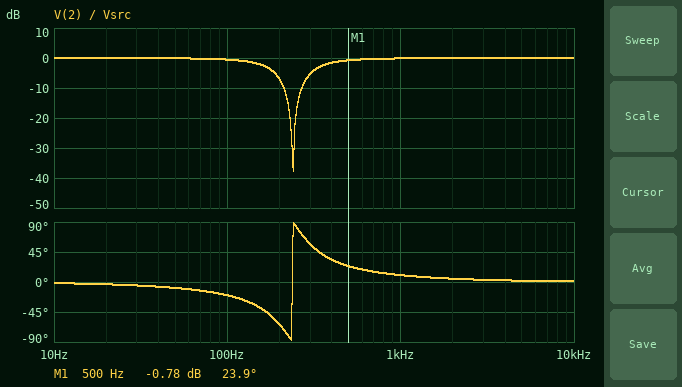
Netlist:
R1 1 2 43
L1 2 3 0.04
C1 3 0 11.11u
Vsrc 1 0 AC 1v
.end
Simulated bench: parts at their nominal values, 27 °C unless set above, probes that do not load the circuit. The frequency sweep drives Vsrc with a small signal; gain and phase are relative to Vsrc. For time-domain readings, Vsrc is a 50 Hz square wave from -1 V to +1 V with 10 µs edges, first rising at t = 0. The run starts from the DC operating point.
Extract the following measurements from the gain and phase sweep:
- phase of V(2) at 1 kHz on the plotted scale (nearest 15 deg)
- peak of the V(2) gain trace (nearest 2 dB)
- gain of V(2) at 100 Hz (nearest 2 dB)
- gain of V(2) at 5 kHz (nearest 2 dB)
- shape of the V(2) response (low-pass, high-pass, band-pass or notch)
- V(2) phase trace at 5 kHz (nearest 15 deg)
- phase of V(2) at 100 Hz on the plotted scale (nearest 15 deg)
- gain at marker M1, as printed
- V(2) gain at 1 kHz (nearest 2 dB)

15 deg
0 dB
0 dB
0 dB
notch
0 deg
-15 deg
-0.78 dB
0 dB
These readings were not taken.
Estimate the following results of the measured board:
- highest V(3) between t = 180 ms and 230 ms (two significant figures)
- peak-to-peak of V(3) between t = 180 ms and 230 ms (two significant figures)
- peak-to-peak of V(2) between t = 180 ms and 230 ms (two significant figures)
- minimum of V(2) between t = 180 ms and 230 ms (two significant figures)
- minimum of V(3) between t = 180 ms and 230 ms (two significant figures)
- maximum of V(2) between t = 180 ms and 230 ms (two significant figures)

1.6 V
3.2 V
2.5 V
-1.3 V
-1.6 V
1.3 V
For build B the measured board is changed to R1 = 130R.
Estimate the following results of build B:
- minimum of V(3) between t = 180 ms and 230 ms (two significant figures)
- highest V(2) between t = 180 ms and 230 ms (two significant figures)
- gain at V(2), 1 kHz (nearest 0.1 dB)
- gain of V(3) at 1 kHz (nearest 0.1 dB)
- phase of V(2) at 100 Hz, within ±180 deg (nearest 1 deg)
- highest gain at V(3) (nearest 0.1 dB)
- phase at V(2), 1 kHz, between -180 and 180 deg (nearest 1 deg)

-1.0 V
1.0 V
-1.1 dB
-25.5 dB
-48 deg
0 dB
29 deg
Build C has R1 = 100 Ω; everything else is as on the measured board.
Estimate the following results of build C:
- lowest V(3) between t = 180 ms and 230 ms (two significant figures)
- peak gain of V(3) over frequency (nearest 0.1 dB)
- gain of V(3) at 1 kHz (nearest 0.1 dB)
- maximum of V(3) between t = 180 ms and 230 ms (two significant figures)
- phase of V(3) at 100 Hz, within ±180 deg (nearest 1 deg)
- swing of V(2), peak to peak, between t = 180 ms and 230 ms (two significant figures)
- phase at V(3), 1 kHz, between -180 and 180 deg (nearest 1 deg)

-1.0 V
0 dB
-25.1 dB
1.0 V
-40 deg
2.0 V
-157 deg
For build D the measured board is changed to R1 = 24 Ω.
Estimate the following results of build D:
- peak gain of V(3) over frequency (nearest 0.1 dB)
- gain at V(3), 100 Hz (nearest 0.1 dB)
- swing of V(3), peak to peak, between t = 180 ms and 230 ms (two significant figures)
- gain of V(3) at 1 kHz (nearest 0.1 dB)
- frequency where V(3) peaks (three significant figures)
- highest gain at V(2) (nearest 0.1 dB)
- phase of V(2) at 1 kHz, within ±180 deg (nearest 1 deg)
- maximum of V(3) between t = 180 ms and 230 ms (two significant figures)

8.1 dB
1.5 dB
4.1 V
-24.4 dB
229 Hz
0 dB
6 deg
2.1 V
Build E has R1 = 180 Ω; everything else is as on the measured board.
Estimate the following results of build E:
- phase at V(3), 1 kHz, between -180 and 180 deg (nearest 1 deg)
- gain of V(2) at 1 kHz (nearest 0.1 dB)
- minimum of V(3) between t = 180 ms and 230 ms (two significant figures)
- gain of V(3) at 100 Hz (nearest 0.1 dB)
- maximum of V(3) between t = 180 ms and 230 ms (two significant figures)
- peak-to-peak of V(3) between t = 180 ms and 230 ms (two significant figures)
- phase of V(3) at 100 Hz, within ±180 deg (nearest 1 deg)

-143 deg
-2.0 dB
-990 mV
-3.5 dB
990 mV
2.0 V
-57 deg
